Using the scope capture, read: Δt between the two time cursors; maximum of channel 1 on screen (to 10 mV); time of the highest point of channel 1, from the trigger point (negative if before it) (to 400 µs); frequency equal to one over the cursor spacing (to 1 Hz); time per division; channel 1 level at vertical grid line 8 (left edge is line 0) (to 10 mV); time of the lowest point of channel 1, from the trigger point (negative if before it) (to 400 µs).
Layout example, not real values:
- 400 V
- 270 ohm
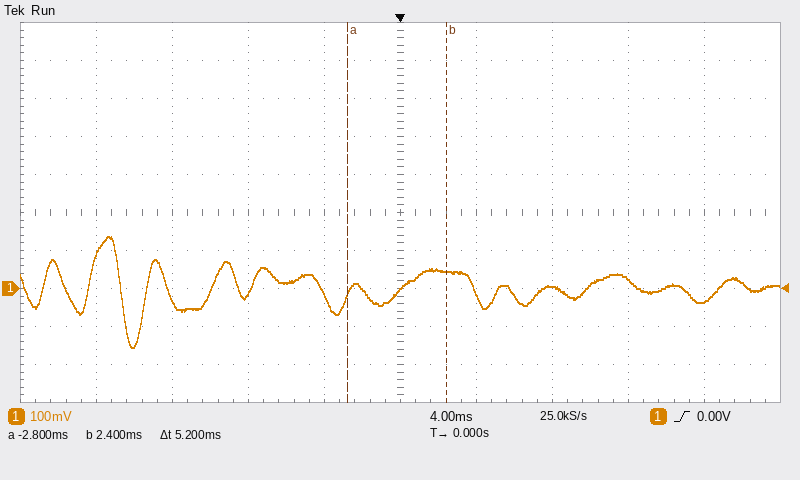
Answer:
- 5.2 ms
- 140 mV
- -15.2 ms
- 192 Hz
- 4 ms
- 20 mV
- -14.0 ms
